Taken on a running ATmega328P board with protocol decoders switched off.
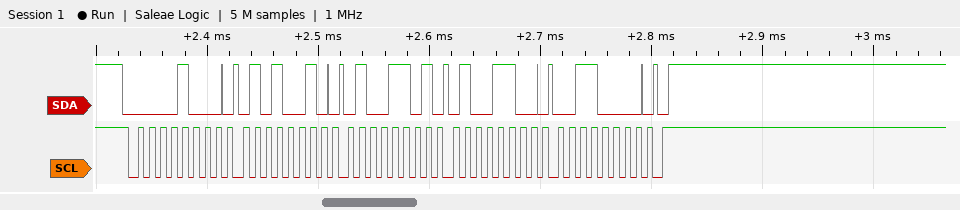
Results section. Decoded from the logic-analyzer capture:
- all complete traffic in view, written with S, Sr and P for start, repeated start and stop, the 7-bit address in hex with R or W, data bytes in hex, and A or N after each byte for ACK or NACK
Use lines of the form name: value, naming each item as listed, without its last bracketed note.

all complete traffic in view, written with S, Sr and P for start, repeated start and stop, the 7-bit address in hex with R or W, data bytes in hex, and A or N after each byte for ACK or NACK: S 04W A 52 A 4D A 4C A 30 A P
